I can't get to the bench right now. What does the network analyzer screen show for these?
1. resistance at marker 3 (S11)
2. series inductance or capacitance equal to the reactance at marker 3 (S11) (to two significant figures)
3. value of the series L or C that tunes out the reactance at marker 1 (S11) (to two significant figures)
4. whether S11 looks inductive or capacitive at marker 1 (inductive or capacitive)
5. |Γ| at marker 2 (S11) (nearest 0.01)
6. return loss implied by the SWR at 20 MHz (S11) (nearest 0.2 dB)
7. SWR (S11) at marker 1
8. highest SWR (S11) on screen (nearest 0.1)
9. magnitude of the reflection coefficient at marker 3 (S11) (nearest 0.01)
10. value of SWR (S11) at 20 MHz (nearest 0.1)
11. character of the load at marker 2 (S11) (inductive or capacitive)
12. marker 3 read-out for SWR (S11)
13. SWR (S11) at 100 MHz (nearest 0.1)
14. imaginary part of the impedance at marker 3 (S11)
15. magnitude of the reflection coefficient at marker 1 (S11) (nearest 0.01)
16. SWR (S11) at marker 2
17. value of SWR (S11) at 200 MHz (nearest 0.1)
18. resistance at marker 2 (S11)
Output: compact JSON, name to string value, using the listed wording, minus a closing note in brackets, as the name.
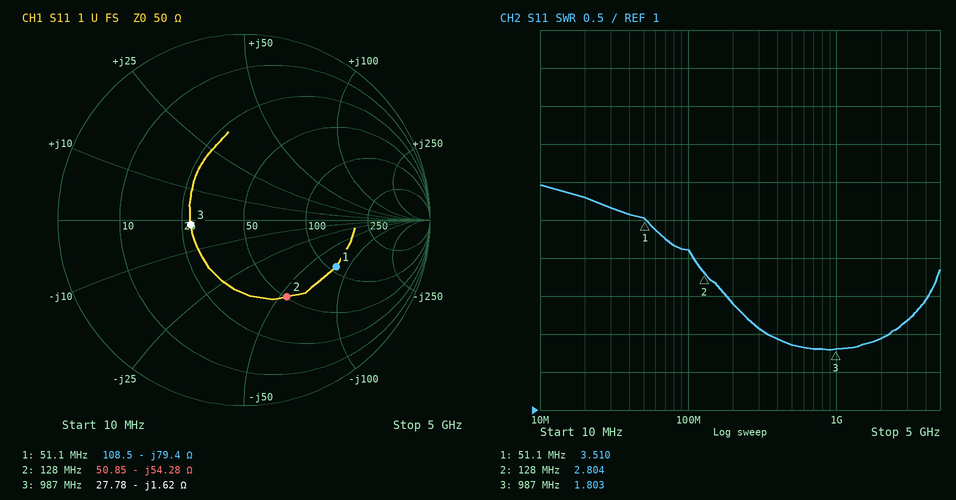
{"resistance at marker 3": "27.78 Ω", "series inductance or capacitance equal to the reactance at marker 3 (S11)": "100 pF", "value of the series L or C that tunes out the reactance at marker 1 (S11)": "250 nH", "whether S11 looks inductive or capacitive at marker 1": "capacitive", "|Γ| at marker 2 (S11)": "0.47", "return loss implied by the SWR at 20 MHz (S11)": "4.6 dB", "SWR (S11) at marker 1": "3.510", "highest SWR (S11) on screen": "4.0", "magnitude of the reflection coefficient at marker 3 (S11)": "0.29", "value of SWR (S11) at 20 MHz": "3.8", "character of the load at marker 2 (S11)": "capacitive", "marker 3 read-out for SWR": "1.803", "SWR (S11) at 100 MHz": "3.1", "imaginary part of the impedance at marker 3": "-1.62 Ω", "magnitude of the reflection coefficient at marker 1 (S11)": "0.56", "SWR (S11) at marker 2": "2.804", "value of SWR (S11) at 200 MHz": "2.4", "resistance at marker 2": "50.85 Ω"}
